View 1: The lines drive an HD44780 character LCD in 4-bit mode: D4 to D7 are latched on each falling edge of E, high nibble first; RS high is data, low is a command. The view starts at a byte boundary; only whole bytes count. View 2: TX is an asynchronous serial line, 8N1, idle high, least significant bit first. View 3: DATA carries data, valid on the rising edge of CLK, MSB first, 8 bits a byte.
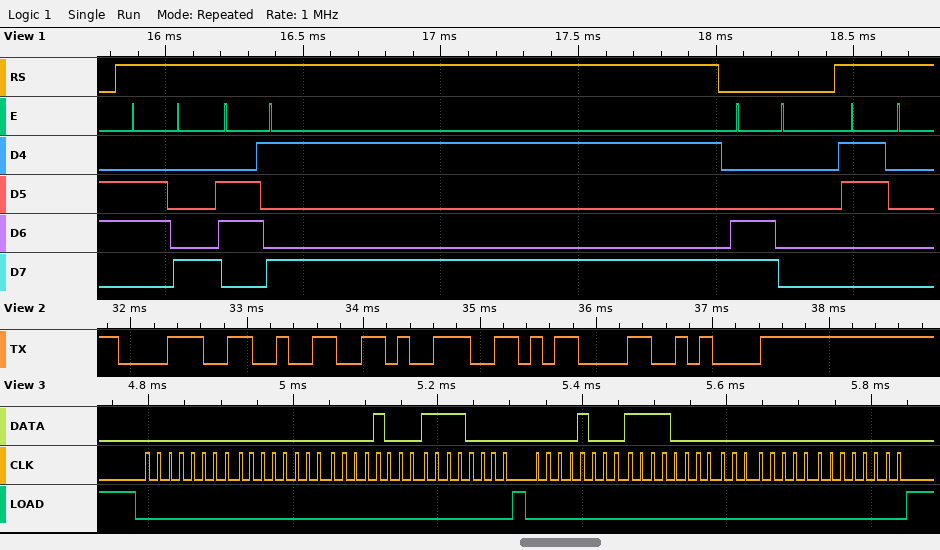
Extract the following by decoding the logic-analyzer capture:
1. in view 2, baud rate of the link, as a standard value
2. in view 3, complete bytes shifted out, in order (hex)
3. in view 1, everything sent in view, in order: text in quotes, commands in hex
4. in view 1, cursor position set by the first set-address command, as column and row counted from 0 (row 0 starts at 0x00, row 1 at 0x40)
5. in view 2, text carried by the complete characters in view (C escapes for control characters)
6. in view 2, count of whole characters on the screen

9600 baud
0x00 0x00 0x08 0xF0 0x08 0xF0 0x00 0x00
"hi" 0xC0 "0"
column 0, row 1
"829\r\n"
5
